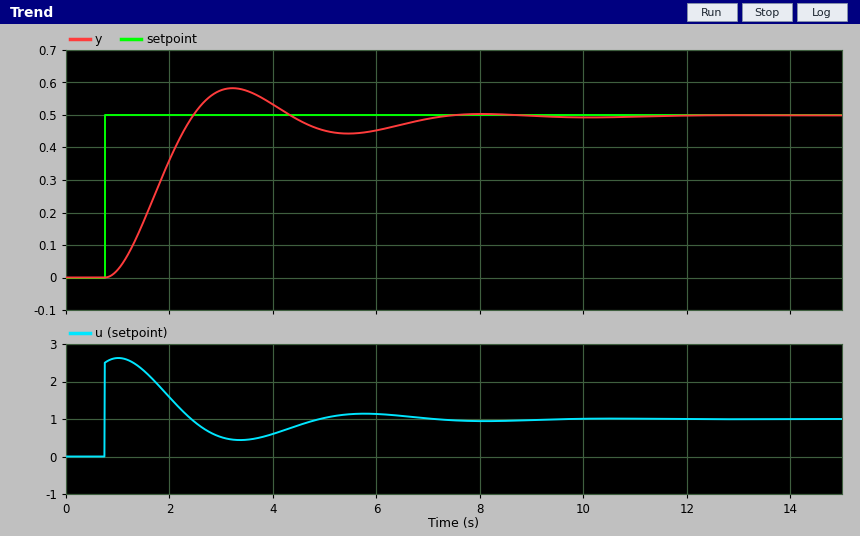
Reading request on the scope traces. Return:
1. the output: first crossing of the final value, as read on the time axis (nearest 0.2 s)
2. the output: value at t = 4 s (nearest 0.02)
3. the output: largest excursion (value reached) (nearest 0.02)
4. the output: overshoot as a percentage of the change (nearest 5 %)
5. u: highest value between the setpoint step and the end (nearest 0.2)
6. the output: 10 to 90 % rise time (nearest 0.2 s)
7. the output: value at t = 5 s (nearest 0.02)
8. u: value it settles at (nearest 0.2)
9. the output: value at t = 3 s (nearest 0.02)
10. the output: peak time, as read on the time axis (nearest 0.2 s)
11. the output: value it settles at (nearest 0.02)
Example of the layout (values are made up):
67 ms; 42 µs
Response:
2.4 s; 0.54; 0.58; 15 %; 2.6; 1.2 s; 0.46; 1.0; 0.58; 3.2 s; 0.50
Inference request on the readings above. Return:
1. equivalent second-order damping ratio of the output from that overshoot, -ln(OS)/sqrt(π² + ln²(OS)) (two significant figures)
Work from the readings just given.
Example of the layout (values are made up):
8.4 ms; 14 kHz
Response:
0.52
